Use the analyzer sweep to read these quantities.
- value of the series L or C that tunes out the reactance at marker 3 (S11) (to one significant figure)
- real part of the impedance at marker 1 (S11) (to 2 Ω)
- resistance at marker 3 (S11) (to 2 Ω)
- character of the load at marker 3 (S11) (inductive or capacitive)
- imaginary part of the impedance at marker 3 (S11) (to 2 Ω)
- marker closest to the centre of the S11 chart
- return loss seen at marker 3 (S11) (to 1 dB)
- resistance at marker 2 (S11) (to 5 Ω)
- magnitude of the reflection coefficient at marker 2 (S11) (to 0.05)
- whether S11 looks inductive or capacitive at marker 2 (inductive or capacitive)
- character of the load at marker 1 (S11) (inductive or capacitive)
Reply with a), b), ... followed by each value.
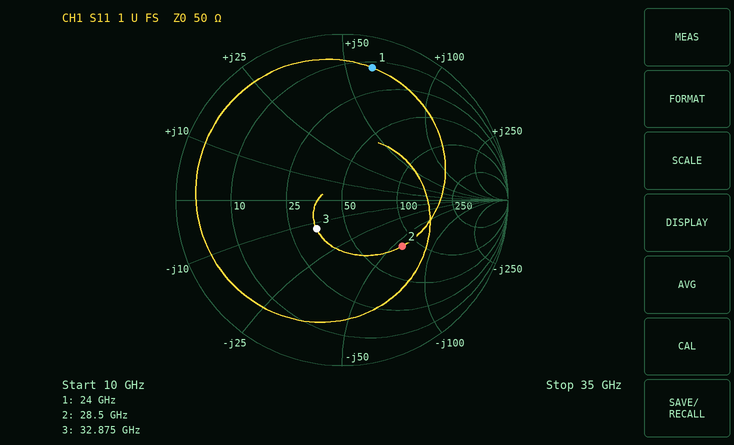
a) 60 pH
b) 12 Ω
c) 34 Ω
d) capacitive
e) -12 Ω
f) marker 3
g) 13 dB
h) 80 Ω
i) 0.45
j) capacitive
k) inductive
